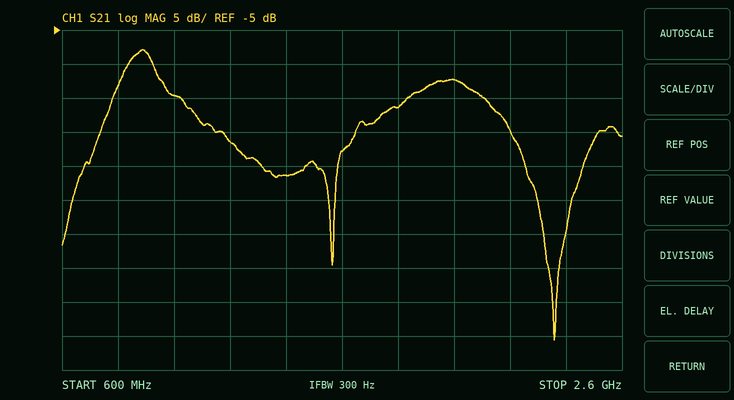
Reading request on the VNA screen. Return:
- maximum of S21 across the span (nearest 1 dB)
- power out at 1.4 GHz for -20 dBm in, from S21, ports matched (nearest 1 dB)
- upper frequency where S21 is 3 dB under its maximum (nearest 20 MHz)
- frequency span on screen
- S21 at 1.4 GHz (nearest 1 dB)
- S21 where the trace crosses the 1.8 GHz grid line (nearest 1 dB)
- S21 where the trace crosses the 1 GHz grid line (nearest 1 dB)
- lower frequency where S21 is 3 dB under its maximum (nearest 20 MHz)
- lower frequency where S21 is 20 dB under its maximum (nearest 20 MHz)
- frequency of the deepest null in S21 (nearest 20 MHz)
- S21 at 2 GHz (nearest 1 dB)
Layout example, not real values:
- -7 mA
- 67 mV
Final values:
- -8 dB
- -46 dBm
- 940 MHz
- 2 GHz
- -26 dB
- -16 dB
- -15 dB
- 820 MHz
- 660 MHz
- 2.36 GHz
- -12 dB
